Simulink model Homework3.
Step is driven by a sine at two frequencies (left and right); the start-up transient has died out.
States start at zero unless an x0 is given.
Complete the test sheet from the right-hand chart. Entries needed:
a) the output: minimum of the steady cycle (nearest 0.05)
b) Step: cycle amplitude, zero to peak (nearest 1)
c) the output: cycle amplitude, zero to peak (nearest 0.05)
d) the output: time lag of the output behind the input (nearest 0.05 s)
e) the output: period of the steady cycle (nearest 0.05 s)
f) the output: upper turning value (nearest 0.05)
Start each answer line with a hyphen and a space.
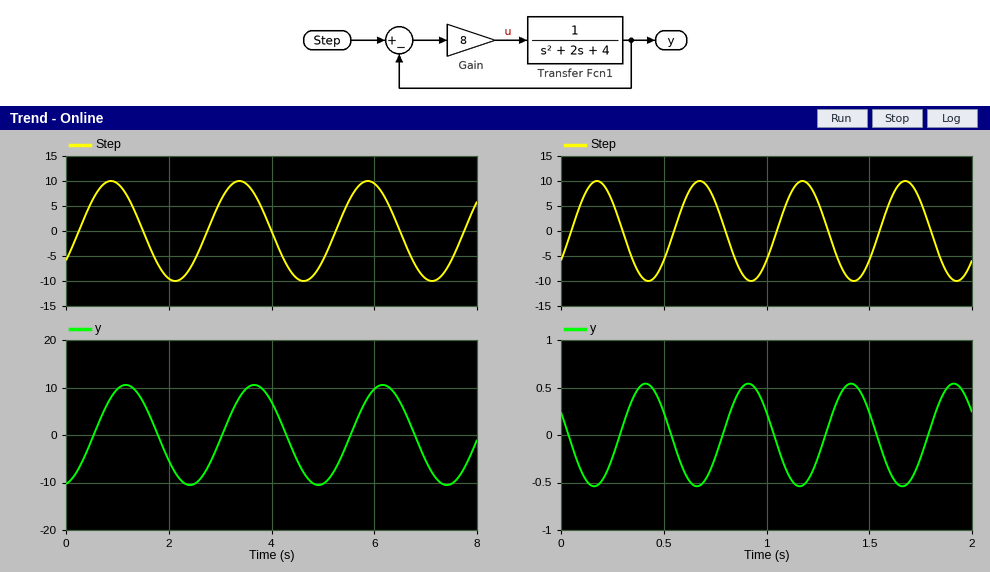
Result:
- -0.55
- 10
- 0.55
- 0.25 s
- 0.50 s
- 0.55
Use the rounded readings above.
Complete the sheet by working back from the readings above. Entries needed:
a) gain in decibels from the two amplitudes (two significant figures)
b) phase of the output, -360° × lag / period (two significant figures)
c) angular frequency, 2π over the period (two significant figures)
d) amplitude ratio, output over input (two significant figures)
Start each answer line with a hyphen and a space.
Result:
- -25 dB
- -180°
- 13 rad/s
- 0.055
